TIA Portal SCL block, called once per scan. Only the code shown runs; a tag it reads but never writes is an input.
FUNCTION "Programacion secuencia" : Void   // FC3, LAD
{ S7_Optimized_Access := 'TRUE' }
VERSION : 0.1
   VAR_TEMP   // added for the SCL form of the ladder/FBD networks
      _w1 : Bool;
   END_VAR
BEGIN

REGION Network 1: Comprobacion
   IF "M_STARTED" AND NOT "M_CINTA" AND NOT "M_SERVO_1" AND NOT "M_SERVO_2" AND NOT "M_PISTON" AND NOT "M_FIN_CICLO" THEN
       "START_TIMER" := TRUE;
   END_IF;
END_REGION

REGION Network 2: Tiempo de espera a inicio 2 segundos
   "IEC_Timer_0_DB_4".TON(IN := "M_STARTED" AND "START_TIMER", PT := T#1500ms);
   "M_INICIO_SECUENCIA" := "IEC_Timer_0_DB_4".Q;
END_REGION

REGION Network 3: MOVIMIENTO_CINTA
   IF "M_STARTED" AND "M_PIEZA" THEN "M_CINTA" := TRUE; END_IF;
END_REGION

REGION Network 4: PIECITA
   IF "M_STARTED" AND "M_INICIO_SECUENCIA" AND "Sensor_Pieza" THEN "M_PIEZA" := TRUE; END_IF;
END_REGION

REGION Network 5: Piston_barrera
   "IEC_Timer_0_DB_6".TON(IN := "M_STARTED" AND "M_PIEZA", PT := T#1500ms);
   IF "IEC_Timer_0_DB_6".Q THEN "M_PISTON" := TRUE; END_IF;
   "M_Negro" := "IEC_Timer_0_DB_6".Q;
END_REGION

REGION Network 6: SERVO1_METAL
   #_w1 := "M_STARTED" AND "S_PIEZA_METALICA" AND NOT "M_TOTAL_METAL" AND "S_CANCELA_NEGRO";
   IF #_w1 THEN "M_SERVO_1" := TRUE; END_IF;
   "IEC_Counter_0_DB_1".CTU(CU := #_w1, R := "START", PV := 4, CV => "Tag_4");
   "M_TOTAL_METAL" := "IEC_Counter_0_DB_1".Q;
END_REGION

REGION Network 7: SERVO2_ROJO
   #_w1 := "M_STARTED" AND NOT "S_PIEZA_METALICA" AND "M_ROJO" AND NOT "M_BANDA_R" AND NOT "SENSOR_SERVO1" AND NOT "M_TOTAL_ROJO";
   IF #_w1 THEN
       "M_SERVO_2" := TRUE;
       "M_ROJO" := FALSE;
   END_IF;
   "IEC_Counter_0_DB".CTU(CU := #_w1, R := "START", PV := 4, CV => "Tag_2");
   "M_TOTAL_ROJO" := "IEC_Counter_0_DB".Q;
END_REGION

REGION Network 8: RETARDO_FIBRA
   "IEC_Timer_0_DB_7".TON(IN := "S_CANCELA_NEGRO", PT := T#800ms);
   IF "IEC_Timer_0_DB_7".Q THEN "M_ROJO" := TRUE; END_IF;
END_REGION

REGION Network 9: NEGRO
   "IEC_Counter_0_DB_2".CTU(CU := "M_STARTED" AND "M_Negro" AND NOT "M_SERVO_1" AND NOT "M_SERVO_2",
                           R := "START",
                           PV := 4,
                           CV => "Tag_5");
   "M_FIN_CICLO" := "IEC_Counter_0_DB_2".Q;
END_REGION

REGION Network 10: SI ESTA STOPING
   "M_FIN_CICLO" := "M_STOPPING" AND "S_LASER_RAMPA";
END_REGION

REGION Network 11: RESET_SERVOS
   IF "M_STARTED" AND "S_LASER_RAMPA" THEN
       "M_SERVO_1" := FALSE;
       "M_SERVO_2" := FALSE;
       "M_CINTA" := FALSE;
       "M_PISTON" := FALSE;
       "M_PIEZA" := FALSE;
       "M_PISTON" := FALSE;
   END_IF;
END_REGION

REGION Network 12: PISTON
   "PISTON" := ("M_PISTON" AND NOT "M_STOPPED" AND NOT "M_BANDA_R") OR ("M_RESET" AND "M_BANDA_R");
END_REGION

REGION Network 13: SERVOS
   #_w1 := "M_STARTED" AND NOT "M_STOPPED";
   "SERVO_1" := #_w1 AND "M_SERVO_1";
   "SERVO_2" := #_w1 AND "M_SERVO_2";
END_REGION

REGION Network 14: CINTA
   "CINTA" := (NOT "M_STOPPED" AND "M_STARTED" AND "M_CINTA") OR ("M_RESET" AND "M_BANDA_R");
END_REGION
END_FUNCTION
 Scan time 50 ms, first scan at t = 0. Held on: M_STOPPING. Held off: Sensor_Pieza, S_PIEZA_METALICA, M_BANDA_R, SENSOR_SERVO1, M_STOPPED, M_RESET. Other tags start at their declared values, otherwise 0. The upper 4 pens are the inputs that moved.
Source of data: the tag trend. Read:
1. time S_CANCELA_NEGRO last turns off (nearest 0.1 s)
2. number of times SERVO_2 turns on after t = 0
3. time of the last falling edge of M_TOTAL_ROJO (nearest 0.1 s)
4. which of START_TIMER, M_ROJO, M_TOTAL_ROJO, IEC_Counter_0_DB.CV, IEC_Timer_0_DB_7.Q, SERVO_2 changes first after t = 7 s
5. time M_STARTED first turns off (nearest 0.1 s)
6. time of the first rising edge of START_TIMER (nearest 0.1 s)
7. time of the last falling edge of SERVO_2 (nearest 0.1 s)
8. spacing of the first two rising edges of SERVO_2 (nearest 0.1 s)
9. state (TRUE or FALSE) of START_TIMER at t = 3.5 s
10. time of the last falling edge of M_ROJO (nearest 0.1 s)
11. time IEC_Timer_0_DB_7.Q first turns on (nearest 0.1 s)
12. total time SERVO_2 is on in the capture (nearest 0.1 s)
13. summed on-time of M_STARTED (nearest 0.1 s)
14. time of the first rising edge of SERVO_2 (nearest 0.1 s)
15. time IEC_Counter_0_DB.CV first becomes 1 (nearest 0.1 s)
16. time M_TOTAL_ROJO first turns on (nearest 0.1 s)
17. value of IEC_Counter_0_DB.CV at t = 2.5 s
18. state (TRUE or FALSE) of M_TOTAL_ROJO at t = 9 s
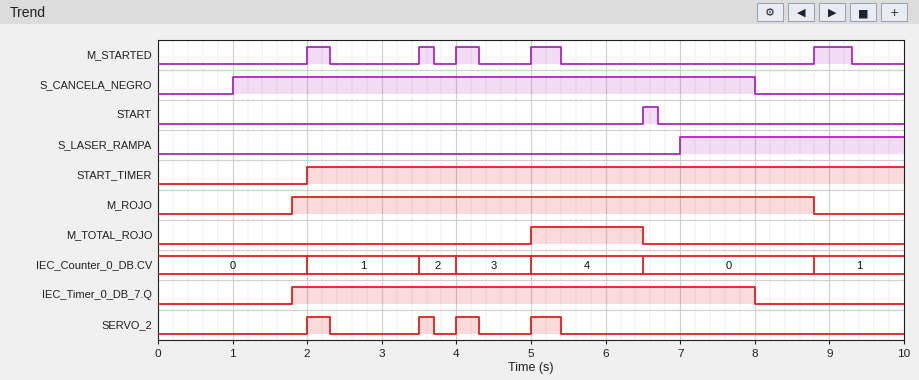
8.0 s
4
6.5 s
IEC_Timer_0_DB_7.Q
2.3 s
2.0 s
5.4 s
1.5 s
TRUE
8.8 s
1.8 s
1.2 s
1.7 s
2.0 s
2.0 s
5.0 s
1
FALSE
